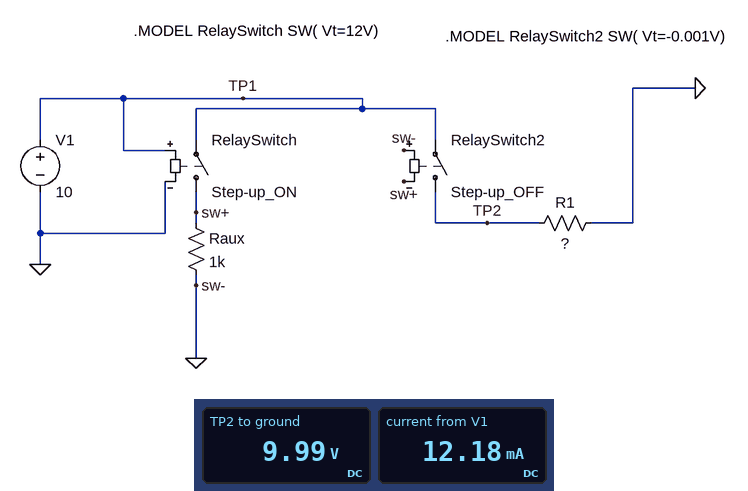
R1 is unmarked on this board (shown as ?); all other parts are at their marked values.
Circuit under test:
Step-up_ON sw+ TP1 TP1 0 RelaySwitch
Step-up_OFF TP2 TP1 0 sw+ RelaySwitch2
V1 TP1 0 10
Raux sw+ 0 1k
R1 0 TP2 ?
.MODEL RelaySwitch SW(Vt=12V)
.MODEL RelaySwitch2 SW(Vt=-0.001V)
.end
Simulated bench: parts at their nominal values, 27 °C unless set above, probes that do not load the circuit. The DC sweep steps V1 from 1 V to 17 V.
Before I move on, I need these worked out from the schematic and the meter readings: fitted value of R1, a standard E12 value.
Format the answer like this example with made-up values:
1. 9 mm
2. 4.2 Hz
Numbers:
1. 820 Ω
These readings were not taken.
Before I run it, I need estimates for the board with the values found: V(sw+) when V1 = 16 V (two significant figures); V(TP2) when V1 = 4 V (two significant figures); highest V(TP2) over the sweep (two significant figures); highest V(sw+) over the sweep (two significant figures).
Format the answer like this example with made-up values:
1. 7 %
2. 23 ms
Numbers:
1. 16 V
2. 4.0 V
3. 12 V
4. 17 V
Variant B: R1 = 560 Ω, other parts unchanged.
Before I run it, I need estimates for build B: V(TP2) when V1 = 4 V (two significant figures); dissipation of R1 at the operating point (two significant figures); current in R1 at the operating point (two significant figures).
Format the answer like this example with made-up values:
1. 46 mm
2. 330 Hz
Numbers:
1. 4.0 V
2. 180 mW
3. 18 mA
